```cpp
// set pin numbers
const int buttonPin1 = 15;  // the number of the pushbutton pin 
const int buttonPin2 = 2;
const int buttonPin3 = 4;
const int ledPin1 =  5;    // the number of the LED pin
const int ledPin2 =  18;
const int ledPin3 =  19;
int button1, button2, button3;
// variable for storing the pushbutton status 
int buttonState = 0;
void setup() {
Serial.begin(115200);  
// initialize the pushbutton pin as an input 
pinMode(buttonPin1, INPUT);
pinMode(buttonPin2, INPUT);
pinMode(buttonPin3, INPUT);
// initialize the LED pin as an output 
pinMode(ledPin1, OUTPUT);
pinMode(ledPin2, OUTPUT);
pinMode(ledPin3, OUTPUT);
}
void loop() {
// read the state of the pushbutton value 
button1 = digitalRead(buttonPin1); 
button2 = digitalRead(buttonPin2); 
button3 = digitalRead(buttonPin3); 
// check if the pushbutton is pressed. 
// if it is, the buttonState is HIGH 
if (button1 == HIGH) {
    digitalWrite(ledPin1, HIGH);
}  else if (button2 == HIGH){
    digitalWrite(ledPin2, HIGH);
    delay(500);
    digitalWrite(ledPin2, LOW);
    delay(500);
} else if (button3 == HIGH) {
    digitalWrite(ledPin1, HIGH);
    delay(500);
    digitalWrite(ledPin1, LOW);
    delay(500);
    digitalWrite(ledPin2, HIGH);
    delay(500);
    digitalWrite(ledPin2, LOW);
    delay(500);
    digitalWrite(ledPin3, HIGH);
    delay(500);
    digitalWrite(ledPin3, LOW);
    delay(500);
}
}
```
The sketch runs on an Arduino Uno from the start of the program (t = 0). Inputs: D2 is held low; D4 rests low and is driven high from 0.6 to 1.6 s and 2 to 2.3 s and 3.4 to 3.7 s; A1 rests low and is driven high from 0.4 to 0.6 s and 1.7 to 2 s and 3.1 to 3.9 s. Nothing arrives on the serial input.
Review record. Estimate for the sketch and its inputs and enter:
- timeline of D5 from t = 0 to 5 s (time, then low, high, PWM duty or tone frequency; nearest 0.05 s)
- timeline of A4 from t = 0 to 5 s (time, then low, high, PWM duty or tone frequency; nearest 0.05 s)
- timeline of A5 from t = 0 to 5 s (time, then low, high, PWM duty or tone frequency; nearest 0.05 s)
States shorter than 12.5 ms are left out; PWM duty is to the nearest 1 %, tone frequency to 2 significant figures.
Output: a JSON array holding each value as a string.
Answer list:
["0 s low; 0.4 s high; 1.1 s low; 3.6 s high", "0 s low; 1.6 s high; 2.1 s low", "0 s low; 2.6 s high; 3.1 s low"]
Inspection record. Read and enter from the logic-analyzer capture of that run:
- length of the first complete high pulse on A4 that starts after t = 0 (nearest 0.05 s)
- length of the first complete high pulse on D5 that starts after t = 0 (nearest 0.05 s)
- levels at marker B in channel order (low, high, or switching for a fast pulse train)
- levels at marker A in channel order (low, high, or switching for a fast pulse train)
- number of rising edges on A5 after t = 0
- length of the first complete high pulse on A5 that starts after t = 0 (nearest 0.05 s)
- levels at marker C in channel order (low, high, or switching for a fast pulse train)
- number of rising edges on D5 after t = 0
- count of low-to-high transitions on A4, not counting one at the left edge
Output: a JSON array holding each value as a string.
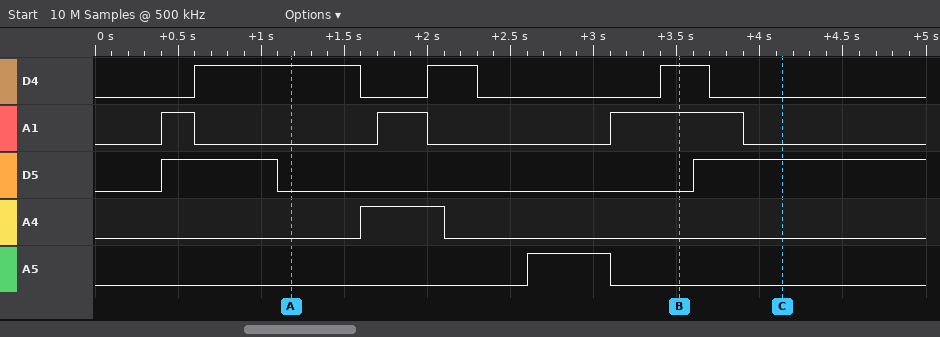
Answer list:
["0.50 s", "0.70 s", "D4 high, A1 high, D5 low, A4 low, A5 low", "D4 high, A1 low, D5 low, A4 low, A5 low", "1", "0.50 s", "D4 low, A1 low, D5 high, A4 low, A5 low", "2", "1"]
